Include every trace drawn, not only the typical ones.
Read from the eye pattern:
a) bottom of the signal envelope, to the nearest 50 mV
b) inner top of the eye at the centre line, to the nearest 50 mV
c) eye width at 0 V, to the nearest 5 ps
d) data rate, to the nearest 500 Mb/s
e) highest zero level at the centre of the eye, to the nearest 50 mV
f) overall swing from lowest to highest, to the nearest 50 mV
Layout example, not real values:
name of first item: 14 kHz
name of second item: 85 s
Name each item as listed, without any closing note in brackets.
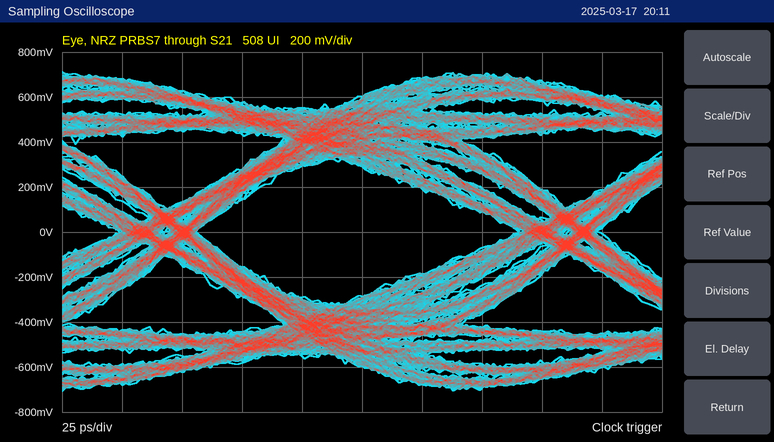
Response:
bottom of the signal envelope, to the nearest 50 mV: -700 mV
inner top of the eye at the centre line, to the nearest 50 mV: 300 mV
eye width at 0 V, to the nearest 5 ps: 135 ps
data rate, to the nearest 500 Mb/s: 6.0 Gb/s
highest zero level at the centre of the eye, to the nearest 50 mV: -300 mV
overall swing from lowest to highest, to the nearest 50 mV: 1.40 V
